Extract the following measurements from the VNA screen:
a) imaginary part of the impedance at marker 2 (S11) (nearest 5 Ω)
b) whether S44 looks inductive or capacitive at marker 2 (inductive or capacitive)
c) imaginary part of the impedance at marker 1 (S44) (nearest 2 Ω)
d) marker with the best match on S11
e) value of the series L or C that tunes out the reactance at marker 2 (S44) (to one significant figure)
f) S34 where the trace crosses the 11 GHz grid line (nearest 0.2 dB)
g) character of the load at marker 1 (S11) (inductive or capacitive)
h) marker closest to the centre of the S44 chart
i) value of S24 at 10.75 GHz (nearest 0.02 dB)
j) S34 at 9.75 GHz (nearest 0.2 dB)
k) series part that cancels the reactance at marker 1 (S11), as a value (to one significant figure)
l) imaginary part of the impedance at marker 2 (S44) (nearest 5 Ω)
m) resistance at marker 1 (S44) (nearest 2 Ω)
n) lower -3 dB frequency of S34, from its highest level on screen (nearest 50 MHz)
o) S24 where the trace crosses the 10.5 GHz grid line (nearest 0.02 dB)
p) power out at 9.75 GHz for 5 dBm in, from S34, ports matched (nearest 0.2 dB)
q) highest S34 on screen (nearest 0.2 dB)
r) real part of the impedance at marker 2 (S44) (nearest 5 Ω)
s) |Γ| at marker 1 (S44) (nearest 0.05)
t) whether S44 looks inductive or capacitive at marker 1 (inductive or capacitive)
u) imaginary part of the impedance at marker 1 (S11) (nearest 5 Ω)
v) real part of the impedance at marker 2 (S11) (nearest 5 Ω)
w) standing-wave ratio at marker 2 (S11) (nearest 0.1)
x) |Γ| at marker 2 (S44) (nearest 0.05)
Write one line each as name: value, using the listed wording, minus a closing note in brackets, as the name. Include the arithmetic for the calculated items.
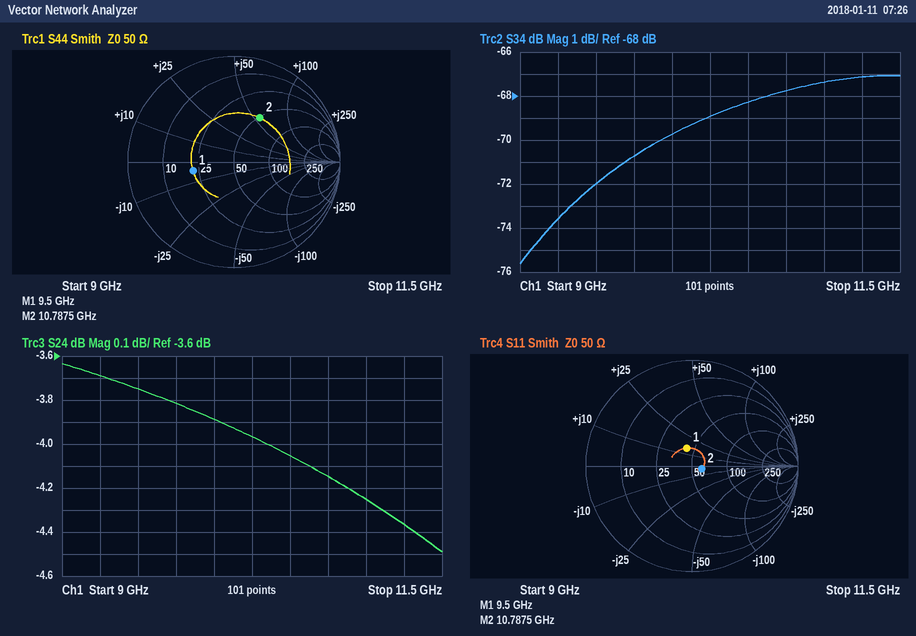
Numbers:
imaginary part of the impedance at marker 2 (S11): -5 Ω
whether S44 looks inductive or capacitive at marker 2: inductive
imaginary part of the impedance at marker 1 (S44): -4 Ω
marker with the best match on S11: marker 2
value of the series L or C that tunes out the reactance at marker 2 (S44): C = 1/(2π × 10.7875 GHz × 55 Ω) ≈ 268 fF, so 300 fF to one significant figure
S34 where the trace crosses the 11 GHz grid line: -67.4 dB
character of the load at marker 1 (S11): inductive
marker closest to the centre of the S44 chart: marker 1
value of S24 at 10.75 GHz: -4.14 dB
S34 at 9.75 GHz: -70.8 dB
series part that cancels the reactance at marker 1 (S11), as a value: C = 1/(2π × 9.5 GHz × 15 Ω) ≈ 1 pF
imaginary part of the impedance at marker 2 (S44): +55 Ω
resistance at marker 1 (S44): 22 Ω
lower -3 dB frequency of S34, from its highest level on screen: 9.90 GHz
S24 where the trace crosses the 10.5 GHz grid line: -4.06 dB
power out at 9.75 GHz for 5 dBm in, from S34, ports matched: 5 dBm + (-70.8 dB) = -65.8 dBm
highest S34 on screen: -67.0 dB
real part of the impedance at marker 2 (S44): 50 Ω
|Γ| at marker 1 (S44): 0.40
whether S44 looks inductive or capacitive at marker 1: capacitive
imaginary part of the impedance at marker 1 (S11): +15 Ω
real part of the impedance at marker 2 (S11): 60 Ω
standing-wave ratio at marker 2 (S11): 1.2
|Γ| at marker 2 (S44): 0.50
